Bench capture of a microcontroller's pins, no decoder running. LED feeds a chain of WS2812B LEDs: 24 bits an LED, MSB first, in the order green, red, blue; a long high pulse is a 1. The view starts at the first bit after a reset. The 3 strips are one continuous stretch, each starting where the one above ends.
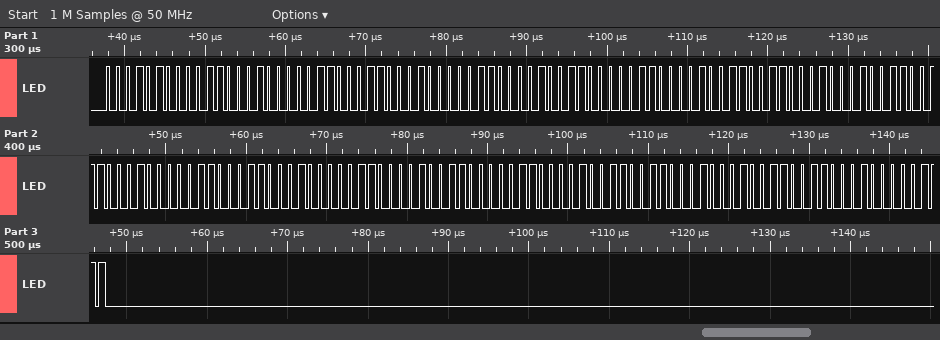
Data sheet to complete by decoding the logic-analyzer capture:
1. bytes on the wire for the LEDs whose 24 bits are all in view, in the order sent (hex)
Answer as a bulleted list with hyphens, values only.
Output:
- 14 31 06 31 06 13 06 13 31 13 31 06 31 06 13 06 13 31 13 31 07
